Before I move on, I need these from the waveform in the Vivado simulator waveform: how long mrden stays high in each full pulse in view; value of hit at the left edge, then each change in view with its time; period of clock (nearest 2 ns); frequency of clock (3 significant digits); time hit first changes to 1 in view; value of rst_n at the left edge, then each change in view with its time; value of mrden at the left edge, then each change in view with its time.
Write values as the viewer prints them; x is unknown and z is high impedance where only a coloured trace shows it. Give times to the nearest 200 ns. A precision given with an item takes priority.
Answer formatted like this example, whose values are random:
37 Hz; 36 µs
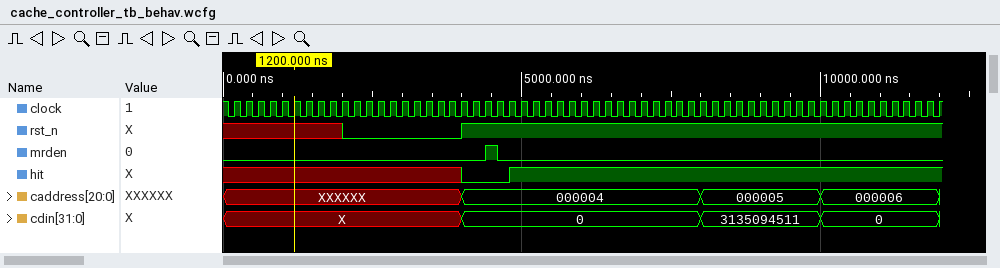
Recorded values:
200 ns; x, 0 at 4000 ns, 1 at 4800 ns; 200 ns; 5.00 MHz; 4800 ns; x, 0 at 2000 ns, 1 at 4000 ns; 0, 1 at 4400 ns, 0 at 4600 ns
